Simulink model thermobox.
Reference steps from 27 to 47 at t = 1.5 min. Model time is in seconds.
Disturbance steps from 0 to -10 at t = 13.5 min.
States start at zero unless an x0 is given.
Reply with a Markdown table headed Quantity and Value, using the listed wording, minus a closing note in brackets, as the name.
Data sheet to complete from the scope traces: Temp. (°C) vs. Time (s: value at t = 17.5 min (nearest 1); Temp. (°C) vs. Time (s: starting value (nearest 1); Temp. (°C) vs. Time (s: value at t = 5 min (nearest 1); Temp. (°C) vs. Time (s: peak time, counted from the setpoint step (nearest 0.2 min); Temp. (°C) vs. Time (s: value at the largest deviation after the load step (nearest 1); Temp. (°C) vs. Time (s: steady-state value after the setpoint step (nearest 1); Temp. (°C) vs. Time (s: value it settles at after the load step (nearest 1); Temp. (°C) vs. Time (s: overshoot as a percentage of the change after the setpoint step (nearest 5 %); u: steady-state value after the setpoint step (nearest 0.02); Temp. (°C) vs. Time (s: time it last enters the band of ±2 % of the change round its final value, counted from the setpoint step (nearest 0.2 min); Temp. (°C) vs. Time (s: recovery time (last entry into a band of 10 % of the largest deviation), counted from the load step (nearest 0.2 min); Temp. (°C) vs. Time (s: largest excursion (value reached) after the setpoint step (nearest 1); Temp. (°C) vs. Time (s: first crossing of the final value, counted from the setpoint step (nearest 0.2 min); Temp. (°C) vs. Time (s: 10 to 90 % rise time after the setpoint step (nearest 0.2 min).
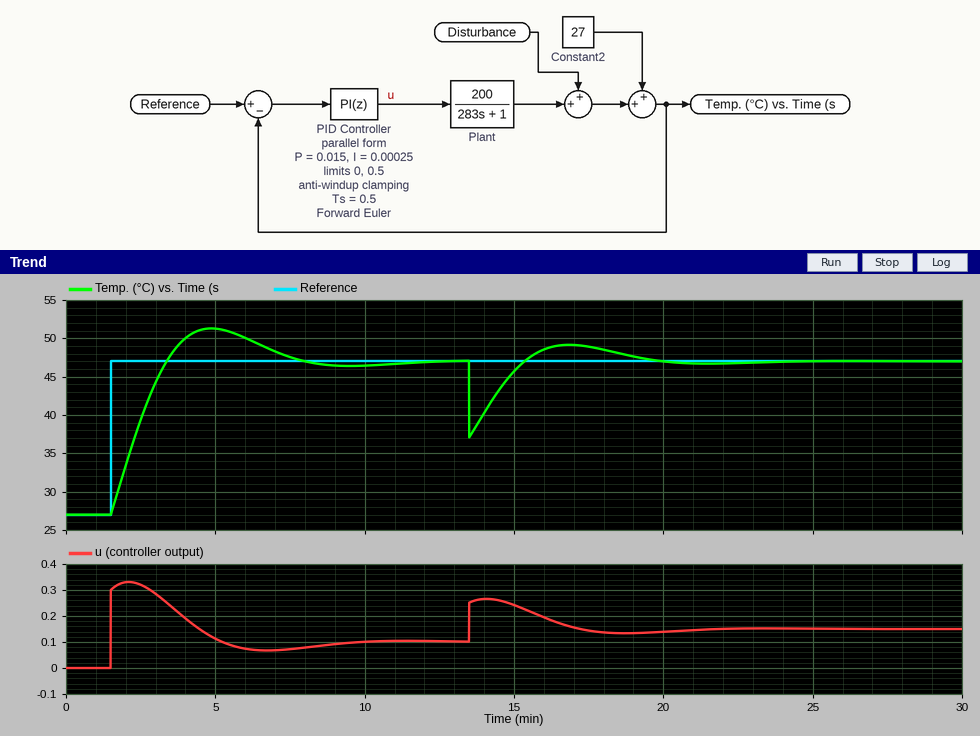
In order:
| Quantity | Value |
|---|---|
| Temp. (°C) vs. Time (s: value at t = 17.5 min | 49 |
| Temp. (°C) vs. Time (s: starting value | 27 |
| Temp. (°C) vs. Time (s: value at t = 5 min | 51 |
| Temp. (°C) vs. Time (s: peak time, counted from the setpoint step | 3.4 min |
| Temp. (°C) vs. Time (s: value at the largest deviation after the load step | 37 |
| Temp. (°C) vs. Time (s: steady-state value after the setpoint step | 47 |
| Temp. (°C) vs. Time (s: value it settles at after the load step | 47 |
| Temp. (°C) vs. Time (s: overshoot as a percentage of the change after the setpoint step | 20 % |
| u: steady-state value after the setpoint step | 0.10 |
| Temp. (°C) vs. Time (s: time it last enters the band of ±2 % of the change round its final value, counted from the setpoint step | 9.2 min |
| Temp. (°C) vs. Time (s: recovery time (last entry into a band of 10 % of the largest deviation), counted from the load step | 5.0 min |
| Temp. (°C) vs. Time (s: largest excursion (value reached) after the setpoint step | 51 |
| Temp. (°C) vs. Time (s: first crossing of the final value, counted from the setpoint step | 1.8 min |
| Temp. (°C) vs. Time (s: 10 to 90 % rise time after the setpoint step | 1.4 min |
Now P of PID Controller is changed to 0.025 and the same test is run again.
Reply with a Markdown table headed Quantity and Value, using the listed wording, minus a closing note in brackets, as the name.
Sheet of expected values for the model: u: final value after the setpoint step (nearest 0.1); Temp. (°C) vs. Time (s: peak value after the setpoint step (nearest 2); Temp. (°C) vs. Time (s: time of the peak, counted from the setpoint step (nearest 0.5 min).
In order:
| Quantity | Value |
|---|---|
| u: final value after the setpoint step | 0.1 |
| Temp. (°C) vs. Time (s: peak value after the setpoint step | 50 |
| Temp. (°C) vs. Time (s: time of the peak, counted from the setpoint step | 3.0 min |
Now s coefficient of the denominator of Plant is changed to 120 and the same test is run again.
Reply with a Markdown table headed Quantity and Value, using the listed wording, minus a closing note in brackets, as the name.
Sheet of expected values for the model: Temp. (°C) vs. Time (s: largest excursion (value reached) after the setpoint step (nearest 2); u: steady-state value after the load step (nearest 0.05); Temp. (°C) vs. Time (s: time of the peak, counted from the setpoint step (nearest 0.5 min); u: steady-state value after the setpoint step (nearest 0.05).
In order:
| Quantity | Value |
|---|---|
| Temp. (°C) vs. Time (s: largest excursion (value reached) after the setpoint step | 48 |
| u: steady-state value after the load step | 0.15 |
| Temp. (°C) vs. Time (s: time of the peak, counted from the setpoint step | 2.0 min |
| u: steady-state value after the setpoint step | 0.10 |
